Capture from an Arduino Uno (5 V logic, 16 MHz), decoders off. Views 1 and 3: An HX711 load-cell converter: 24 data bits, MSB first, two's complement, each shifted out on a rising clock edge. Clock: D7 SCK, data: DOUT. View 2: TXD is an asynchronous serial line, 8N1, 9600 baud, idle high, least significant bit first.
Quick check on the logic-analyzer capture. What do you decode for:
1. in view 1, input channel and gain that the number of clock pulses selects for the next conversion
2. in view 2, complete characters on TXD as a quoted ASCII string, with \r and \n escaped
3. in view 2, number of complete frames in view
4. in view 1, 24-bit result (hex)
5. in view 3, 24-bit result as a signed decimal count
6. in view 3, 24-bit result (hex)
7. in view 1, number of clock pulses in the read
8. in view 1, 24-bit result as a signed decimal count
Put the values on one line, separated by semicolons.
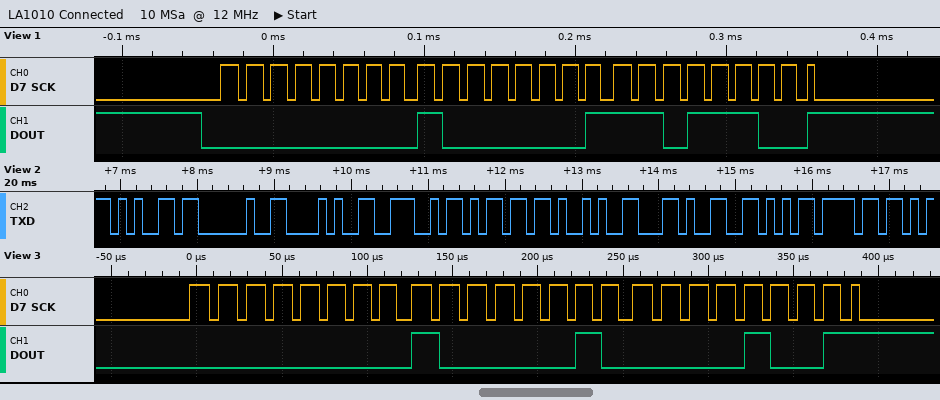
channel A, gain 128; "e (Nm),Vo"; 9; 0x0081DC; 33289; 0x008209; 25; 33244
